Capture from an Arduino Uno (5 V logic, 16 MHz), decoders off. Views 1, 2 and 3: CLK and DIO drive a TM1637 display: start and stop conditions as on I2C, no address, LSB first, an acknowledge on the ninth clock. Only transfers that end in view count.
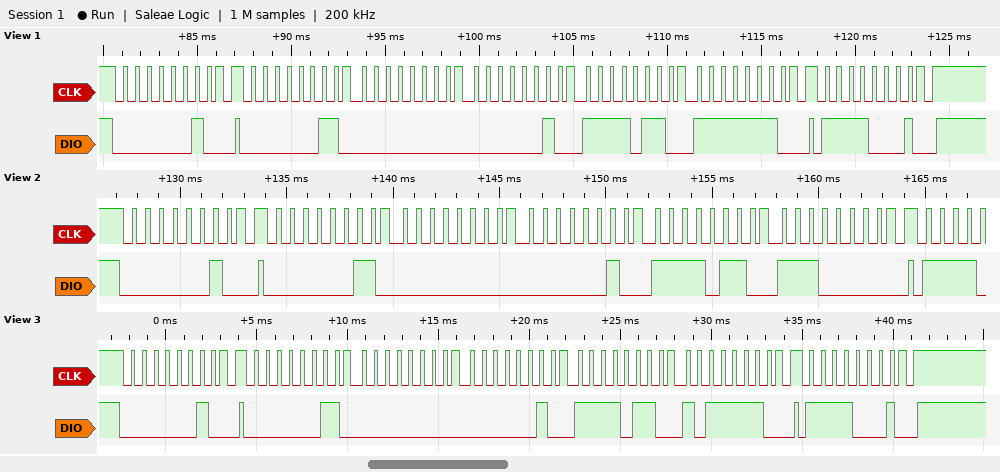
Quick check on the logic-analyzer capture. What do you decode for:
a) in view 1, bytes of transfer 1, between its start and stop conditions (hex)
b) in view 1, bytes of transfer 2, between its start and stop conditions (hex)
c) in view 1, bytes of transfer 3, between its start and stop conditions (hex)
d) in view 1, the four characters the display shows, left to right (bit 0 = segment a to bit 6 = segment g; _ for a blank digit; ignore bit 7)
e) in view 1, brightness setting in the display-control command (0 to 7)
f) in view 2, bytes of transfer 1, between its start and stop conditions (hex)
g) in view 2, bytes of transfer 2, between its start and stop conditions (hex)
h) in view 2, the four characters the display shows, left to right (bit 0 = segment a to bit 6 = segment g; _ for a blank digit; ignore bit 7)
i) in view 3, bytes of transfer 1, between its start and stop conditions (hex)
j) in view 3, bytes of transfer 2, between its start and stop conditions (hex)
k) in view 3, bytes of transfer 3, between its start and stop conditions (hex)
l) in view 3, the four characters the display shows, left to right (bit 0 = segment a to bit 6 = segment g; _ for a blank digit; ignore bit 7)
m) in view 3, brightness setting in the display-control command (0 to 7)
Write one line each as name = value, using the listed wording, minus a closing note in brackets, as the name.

in view 1, bytes of transfer 1, between its start and stop conditions = 40
in view 1, bytes of transfer 2, between its start and stop conditions = C0 00 40 6F 7F
in view 1, bytes of transfer 3, between its start and stop conditions = 8F
in view 1, the four characters the display shows, left to right = _-98
in view 1, brightness setting in the display-control command = 7
in view 2, bytes of transfer 1, between its start and stop conditions = 40
in view 2, bytes of transfer 2, between its start and stop conditions = C0 00 40 6F 07
in view 2, the four characters the display shows, left to right = _-97
in view 3, bytes of transfer 1, between its start and stop conditions = 40
in view 3, bytes of transfer 2, between its start and stop conditions = C0 00 40 6F 7D
in view 3, bytes of transfer 3, between its start and stop conditions = 8F
in view 3, the four characters the display shows, left to right = _-96
in view 3, brightness setting in the display-control command = 7
